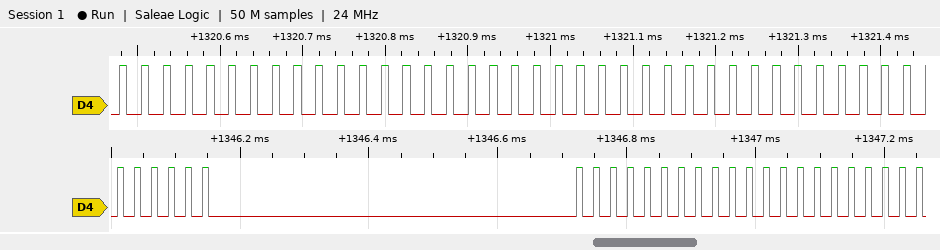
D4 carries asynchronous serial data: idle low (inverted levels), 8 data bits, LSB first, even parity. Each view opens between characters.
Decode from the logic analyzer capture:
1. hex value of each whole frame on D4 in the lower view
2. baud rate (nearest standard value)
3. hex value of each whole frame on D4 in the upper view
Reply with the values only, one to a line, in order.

DB, FB, DB, DB, DB, DB, DB
115200 baud
DB, DB, DB, DB, DB, DB, DB, DB, DB
